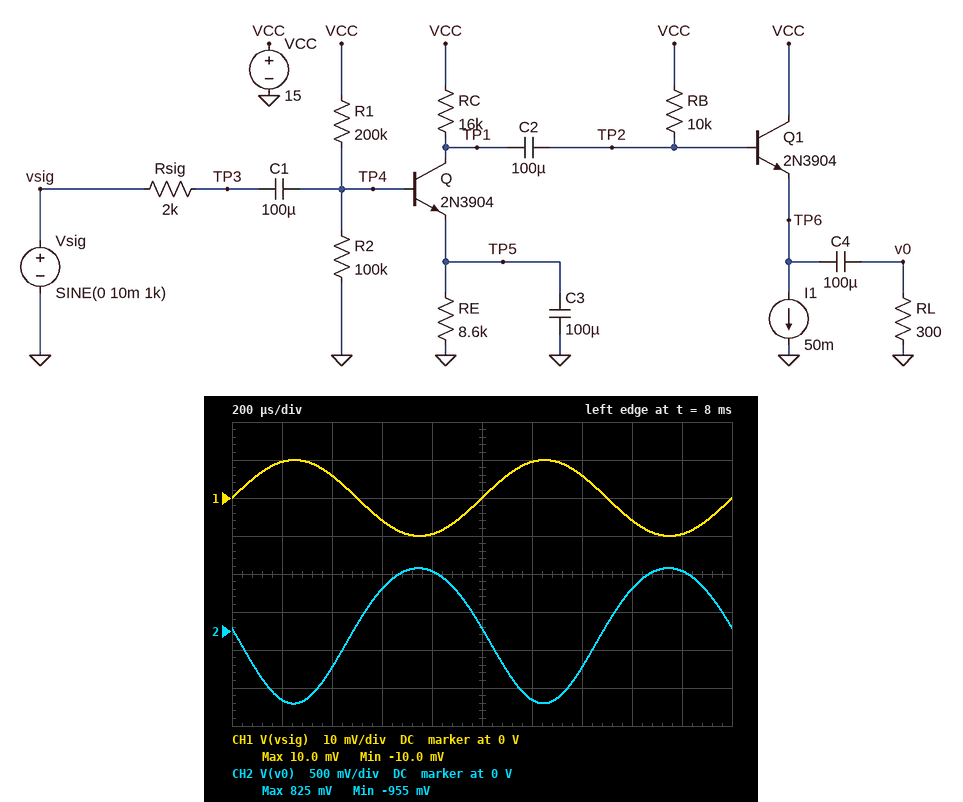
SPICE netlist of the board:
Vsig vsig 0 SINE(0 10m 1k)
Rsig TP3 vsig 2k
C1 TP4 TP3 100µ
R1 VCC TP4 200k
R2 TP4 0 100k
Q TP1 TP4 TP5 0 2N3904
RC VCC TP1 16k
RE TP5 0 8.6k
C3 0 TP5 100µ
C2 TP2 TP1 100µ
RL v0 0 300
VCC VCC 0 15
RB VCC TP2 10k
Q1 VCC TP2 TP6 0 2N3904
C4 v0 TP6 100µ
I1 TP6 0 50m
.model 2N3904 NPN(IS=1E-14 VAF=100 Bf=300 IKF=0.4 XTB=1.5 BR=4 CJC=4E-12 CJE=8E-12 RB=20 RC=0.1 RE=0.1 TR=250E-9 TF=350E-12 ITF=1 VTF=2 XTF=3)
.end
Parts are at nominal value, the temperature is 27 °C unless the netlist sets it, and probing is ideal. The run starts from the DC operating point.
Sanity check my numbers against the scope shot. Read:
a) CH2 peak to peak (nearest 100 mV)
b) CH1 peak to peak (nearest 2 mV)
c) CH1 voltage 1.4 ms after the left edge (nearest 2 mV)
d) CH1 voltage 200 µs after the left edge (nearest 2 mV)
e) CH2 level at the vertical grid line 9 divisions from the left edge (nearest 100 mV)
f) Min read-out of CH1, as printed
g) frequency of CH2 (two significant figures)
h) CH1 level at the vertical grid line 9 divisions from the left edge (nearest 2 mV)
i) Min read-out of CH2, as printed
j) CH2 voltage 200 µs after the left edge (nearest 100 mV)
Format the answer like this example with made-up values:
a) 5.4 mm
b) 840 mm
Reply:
a) 1.8 V
b) 20 mV
c) 6 mV
d) 10 mV
e) 800 mV
f) -10.0 mV
g) 1.0 kHz
h) -10 mV
i) -955 mV
j) -900 mV
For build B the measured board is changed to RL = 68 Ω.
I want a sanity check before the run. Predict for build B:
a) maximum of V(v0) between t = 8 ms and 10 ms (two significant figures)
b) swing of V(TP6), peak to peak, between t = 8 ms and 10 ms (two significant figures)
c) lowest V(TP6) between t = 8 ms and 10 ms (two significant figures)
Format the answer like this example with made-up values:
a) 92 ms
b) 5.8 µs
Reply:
a) 660 mV
b) 1.4 V
c) 12 V
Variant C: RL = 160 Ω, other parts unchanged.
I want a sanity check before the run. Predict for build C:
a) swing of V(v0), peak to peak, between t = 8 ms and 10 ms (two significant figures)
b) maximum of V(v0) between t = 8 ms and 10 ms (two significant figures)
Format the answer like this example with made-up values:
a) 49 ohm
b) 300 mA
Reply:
a) 1.7 V
b) 780 mV
